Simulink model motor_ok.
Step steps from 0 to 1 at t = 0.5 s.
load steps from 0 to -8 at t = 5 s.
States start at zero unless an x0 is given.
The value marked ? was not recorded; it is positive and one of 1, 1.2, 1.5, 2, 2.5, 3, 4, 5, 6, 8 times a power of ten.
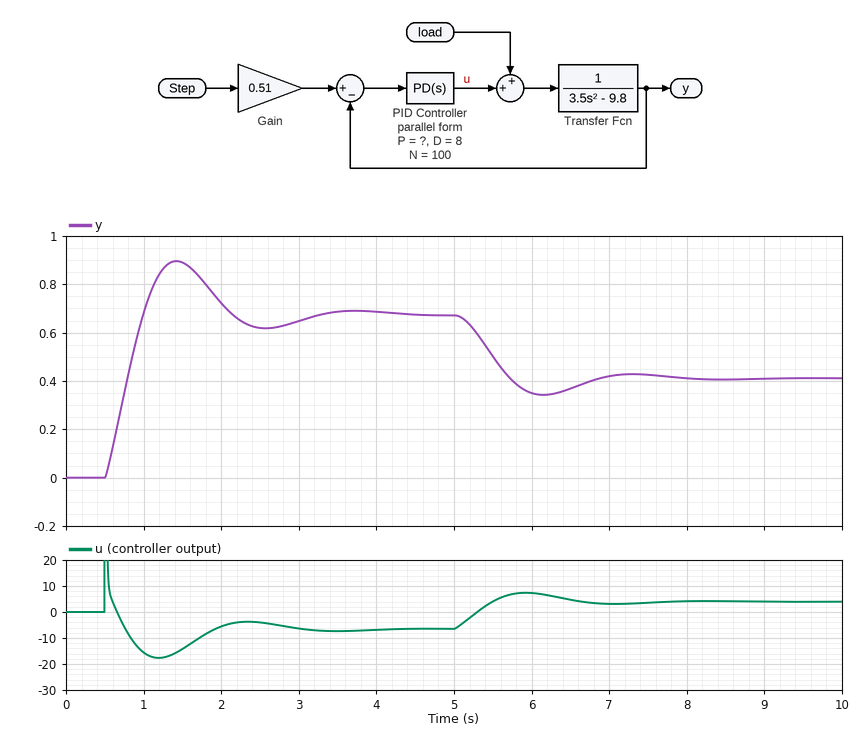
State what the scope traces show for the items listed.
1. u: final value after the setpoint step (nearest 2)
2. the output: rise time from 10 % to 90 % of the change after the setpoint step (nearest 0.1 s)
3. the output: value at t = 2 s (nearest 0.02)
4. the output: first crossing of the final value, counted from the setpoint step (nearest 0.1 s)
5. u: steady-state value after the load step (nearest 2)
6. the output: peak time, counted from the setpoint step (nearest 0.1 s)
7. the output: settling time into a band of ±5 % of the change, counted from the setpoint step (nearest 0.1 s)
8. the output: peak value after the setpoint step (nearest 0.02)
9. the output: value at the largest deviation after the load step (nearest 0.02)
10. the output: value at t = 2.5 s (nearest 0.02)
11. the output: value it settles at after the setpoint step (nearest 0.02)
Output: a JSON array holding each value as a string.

["-6", "0.4 s", "0.72", "0.5 s", "4", "0.9 s", "2.4 s", "0.90", "0.34", "0.62", "0.68"]
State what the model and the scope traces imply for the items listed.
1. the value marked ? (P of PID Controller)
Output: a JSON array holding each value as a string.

["40"]
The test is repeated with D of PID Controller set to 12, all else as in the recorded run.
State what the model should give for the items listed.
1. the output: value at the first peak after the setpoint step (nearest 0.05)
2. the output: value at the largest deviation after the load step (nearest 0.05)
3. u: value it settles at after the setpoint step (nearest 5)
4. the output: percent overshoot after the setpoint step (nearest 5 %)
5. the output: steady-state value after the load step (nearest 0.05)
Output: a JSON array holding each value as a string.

["0.80", "0.40", "-5", "20 %", "0.40"]
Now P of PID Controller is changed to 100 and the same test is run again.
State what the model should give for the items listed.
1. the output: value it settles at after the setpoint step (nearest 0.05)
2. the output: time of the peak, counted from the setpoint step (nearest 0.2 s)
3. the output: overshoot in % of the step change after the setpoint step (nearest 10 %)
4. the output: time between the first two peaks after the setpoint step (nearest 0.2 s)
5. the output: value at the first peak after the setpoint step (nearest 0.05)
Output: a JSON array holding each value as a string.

["0.55", "0.6 s", "50 %", "1.2 s", "0.85"]
